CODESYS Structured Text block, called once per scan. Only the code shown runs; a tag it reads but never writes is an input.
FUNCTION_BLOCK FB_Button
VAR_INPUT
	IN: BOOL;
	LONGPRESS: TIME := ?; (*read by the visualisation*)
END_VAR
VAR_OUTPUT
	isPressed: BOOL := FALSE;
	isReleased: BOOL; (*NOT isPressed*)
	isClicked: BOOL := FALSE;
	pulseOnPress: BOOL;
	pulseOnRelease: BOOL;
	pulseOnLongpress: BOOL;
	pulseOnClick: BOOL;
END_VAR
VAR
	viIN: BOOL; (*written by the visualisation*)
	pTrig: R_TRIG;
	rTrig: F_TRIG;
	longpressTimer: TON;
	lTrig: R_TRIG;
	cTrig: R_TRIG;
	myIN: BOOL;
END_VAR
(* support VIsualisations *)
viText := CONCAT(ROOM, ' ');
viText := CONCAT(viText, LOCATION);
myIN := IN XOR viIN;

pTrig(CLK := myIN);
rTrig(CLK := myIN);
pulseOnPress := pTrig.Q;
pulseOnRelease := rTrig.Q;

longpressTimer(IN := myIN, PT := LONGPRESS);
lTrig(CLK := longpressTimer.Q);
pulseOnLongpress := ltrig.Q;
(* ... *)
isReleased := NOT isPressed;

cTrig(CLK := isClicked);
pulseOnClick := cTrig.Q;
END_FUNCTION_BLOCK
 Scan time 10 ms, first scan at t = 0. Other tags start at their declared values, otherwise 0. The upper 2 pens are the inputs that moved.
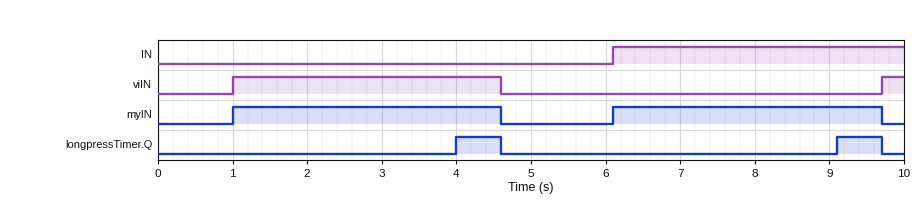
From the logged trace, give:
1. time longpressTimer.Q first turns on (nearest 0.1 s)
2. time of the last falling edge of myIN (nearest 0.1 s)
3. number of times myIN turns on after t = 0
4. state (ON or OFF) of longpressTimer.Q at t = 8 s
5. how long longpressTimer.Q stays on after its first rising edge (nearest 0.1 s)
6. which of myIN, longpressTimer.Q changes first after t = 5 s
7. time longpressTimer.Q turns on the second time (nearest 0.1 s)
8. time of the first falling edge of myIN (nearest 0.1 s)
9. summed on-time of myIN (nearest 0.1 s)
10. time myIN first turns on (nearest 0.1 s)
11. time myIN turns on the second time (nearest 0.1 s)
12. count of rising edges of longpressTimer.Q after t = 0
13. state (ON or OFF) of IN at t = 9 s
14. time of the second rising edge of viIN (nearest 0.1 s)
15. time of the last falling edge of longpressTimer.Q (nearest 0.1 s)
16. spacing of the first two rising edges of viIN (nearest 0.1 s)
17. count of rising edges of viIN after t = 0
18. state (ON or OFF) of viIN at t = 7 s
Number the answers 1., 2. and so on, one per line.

1. 4.0 s
2. 9.7 s
3. 2
4. OFF
5. 0.6 s
6. myIN
7. 9.1 s
8. 4.6 s
9. 7.2 s
10. 1.0 s
11. 6.1 s
12. 2
13. ON
14. 9.7 s
15. 9.7 s
16. 8.7 s
17. 2
18. OFF
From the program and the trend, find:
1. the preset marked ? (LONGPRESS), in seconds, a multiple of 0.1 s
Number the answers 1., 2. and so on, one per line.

1. 3.0 s
